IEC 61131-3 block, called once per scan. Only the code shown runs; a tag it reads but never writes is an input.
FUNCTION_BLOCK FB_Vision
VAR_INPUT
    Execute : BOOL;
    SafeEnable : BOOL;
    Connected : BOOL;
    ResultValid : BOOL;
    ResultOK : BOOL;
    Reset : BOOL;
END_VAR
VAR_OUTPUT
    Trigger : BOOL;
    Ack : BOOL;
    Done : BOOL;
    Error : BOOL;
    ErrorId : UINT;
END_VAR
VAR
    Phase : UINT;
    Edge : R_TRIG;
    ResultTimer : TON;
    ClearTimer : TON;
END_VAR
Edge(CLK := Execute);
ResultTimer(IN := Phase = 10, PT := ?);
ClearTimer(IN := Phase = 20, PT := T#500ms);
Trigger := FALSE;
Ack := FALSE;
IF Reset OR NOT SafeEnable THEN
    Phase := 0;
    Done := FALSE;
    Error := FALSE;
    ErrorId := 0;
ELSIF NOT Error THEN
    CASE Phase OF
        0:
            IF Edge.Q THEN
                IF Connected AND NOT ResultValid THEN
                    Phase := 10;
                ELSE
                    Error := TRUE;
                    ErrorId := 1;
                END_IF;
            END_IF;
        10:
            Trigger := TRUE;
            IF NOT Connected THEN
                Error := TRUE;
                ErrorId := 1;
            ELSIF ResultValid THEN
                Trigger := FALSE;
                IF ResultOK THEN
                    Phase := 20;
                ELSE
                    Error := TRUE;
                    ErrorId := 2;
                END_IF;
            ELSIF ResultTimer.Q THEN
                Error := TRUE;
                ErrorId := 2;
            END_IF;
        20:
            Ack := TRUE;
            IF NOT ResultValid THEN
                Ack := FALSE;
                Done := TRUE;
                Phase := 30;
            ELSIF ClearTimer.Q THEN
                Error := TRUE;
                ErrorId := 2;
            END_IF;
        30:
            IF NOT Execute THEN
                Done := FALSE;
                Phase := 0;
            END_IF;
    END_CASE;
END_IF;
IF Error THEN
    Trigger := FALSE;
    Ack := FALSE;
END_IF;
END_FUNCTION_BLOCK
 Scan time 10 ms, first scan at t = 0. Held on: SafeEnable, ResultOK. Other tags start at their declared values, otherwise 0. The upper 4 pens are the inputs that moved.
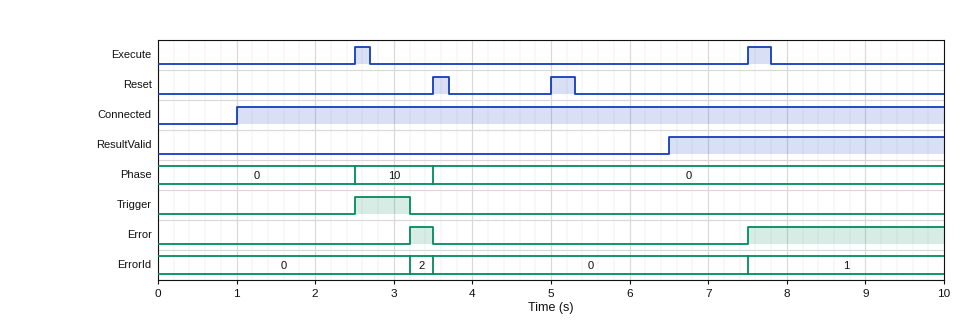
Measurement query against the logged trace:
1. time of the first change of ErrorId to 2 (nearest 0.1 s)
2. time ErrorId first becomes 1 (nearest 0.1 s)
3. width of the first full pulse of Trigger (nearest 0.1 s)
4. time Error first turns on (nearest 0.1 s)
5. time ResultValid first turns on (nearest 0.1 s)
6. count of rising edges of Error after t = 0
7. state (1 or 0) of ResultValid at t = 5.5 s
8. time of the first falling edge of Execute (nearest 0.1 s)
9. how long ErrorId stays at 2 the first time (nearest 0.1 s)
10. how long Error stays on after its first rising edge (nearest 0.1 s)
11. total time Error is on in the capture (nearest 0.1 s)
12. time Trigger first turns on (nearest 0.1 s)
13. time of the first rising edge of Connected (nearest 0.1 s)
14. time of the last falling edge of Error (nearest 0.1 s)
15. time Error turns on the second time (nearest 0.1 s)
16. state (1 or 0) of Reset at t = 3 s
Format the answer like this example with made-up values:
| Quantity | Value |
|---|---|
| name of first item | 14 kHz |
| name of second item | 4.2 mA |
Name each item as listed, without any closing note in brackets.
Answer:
| Quantity | Value |
|---|---|
| time of the first change of ErrorId to 2 | 3.2 s |
| time ErrorId first becomes 1 | 7.5 s |
| width of the first full pulse of Trigger | 0.7 s |
| time Error first turns on | 3.2 s |
| time ResultValid first turns on | 6.5 s |
| count of rising edges of Error after t = 0 | 2 |
| state (1 or 0) of ResultValid at t = 5.5 s | 0 |
| time of the first falling edge of Execute | 2.7 s |
| how long ErrorId stays at 2 the first time | 0.3 s |
| how long Error stays on after its first rising edge | 0.3 s |
| total time Error is on in the capture | 2.8 s |
| time Trigger first turns on | 2.5 s |
| time of the first rising edge of Connected | 1.0 s |
| time of the last falling edge of Error | 3.5 s |
| time Error turns on the second time | 7.5 s |
| state (1 or 0) of Reset at t = 3 s | 0 |
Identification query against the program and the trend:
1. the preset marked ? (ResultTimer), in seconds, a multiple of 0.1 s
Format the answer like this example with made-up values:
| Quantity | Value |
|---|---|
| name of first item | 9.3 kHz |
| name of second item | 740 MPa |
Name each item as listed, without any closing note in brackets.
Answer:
| Quantity | Value |
|---|---|
| the preset marked ? (ResultTimer), in seconds, a multiple of 0.1 s | 0.7 s |
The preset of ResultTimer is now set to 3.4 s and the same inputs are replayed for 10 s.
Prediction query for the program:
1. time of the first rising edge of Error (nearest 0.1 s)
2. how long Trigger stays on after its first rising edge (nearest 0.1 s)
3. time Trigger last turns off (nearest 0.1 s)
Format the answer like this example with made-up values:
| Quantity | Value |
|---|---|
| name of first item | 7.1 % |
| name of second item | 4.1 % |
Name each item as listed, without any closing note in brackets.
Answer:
| Quantity | Value |
|---|---|
| time of the first rising edge of Error | 7.5 s |
| how long Trigger stays on after its first rising edge | 1.0 s |
| time Trigger last turns off | 3.5 s |
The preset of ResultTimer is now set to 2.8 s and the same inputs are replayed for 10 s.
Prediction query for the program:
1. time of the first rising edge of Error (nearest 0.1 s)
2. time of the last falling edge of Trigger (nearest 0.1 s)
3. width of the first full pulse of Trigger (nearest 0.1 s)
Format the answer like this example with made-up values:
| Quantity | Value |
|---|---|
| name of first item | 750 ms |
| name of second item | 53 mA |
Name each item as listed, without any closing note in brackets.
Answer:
| Quantity | Value |
|---|---|
| time of the first rising edge of Error | 7.5 s |
| time of the last falling edge of Trigger | 3.5 s |
| width of the first full pulse of Trigger | 1.0 s |
